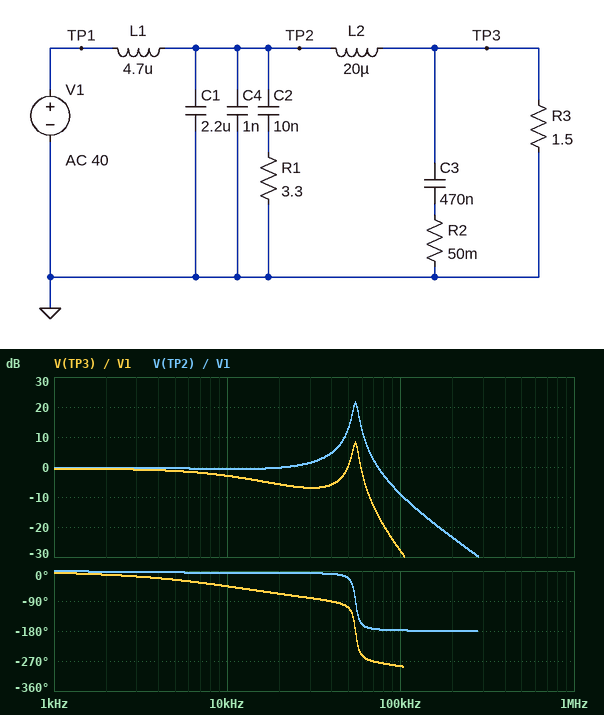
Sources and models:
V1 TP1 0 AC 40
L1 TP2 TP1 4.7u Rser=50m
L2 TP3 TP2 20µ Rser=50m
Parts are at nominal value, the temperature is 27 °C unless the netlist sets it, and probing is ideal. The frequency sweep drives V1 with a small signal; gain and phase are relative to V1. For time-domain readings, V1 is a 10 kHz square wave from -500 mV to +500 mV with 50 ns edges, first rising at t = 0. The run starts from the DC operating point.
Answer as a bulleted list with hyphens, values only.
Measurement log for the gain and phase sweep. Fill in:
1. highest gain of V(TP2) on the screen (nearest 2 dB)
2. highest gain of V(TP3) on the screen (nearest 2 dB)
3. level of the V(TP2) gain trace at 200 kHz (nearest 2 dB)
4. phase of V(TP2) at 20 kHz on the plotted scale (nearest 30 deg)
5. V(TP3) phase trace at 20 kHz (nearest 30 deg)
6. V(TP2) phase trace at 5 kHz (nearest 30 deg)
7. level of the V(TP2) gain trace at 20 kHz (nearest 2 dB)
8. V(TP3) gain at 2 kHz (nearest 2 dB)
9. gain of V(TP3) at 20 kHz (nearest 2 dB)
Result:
- 22 dB
- 8 dB
- -24 dB
- 0 deg
- -60 deg
- 0 deg
- 0 dB
- 0 dB
- -6 dB
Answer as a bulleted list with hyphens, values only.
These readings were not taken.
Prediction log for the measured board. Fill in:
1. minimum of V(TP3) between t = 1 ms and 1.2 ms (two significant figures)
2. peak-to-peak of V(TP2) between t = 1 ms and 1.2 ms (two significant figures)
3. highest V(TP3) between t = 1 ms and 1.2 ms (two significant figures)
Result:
- -520 mV
- 2.1 V
- 520 mV
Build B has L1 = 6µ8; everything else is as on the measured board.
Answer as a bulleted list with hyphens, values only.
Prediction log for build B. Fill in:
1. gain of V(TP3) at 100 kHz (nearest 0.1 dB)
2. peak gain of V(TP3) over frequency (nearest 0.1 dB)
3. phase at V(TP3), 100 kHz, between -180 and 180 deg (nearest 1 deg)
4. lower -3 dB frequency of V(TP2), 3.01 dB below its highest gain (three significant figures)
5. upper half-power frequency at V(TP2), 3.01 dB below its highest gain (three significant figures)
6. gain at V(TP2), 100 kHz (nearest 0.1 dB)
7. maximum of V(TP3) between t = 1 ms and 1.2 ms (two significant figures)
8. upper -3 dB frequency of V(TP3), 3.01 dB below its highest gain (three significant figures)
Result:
- -32.2 dB
- 6.9 dB
- 74 deg
- 45.4 kHz
- 49.5 kHz
- -13.2 dB
- 550 mV
- 49.3 kHz
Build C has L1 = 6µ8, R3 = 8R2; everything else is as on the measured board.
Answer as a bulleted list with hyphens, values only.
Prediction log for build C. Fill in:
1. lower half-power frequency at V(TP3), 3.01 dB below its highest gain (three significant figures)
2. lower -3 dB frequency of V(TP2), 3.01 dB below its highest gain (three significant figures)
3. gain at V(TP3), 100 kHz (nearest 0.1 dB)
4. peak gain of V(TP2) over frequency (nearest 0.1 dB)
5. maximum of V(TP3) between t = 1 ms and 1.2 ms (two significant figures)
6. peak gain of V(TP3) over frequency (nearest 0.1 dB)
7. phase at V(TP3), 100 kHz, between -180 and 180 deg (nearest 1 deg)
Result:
- 29.3 kHz
- 26.8 kHz
- -23.0 dB
- 7.3 dB
- 1.3 V
- 9.8 dB
- 32 deg
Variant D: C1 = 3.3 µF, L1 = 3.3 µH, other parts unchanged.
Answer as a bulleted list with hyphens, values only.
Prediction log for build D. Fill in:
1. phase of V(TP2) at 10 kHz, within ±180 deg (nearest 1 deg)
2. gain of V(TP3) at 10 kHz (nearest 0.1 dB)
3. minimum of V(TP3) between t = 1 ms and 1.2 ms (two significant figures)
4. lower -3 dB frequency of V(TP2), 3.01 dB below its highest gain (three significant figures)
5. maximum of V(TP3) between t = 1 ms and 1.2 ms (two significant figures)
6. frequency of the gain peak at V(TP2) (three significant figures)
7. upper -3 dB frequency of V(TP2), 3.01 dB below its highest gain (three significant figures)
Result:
- -4 deg
- -2.7 dB
- -610 mV
- 50.0 kHz
- 610 mV
- 52.0 kHz
- 53.9 kHz
